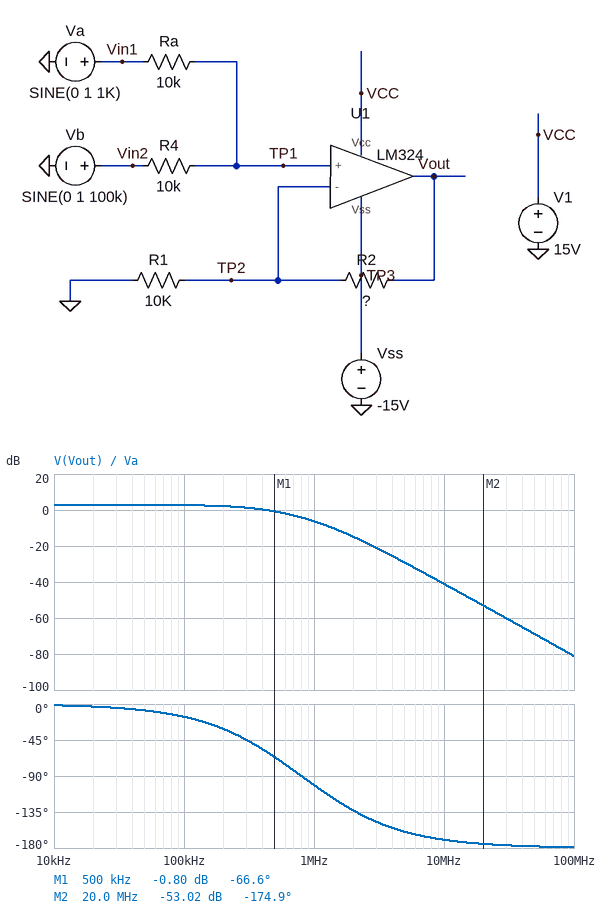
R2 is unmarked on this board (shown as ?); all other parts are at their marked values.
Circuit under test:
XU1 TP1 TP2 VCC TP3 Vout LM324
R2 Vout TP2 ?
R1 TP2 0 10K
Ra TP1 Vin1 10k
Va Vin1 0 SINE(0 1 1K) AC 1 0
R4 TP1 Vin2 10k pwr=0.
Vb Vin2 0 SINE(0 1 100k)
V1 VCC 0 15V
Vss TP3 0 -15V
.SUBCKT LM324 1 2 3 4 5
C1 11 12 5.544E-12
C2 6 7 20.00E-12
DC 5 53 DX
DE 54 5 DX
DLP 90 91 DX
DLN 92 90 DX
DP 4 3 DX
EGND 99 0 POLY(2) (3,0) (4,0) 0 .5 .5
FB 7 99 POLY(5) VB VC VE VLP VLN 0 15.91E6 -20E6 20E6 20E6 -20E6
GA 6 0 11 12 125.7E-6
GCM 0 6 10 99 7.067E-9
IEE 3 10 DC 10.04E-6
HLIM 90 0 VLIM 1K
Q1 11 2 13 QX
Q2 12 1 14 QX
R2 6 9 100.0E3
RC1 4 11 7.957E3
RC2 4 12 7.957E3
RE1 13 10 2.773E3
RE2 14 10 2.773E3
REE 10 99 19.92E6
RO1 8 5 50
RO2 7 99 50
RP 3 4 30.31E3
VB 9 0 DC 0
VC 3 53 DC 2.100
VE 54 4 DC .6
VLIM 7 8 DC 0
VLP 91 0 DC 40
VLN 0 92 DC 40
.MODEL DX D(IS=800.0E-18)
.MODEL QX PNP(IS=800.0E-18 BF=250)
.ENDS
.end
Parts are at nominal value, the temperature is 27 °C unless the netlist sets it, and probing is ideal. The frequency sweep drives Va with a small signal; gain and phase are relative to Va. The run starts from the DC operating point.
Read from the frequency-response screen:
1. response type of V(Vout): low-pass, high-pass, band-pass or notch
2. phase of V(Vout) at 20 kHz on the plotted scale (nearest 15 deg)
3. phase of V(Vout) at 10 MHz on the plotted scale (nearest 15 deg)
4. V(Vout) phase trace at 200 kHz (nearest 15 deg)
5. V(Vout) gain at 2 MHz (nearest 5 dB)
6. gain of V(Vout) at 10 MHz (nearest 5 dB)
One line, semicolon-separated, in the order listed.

low-pass; 0 deg; -165 deg; -30 deg; -15 dB; -40 dB
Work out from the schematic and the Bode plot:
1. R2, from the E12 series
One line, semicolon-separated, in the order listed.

18 kΩ
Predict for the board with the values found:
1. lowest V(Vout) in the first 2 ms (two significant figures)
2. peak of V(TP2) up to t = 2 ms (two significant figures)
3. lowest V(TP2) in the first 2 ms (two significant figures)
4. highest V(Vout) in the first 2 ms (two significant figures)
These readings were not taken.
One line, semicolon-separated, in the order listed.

-2.5 V; 900 mV; -900 mV; 2.5 V
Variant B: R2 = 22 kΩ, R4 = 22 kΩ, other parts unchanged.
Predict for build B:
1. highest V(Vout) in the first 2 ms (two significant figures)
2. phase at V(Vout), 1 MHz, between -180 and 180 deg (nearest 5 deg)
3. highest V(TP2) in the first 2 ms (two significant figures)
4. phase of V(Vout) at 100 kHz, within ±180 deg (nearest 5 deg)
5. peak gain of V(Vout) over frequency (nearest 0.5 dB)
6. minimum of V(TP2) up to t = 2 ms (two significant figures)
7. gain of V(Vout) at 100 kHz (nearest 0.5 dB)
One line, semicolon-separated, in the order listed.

3.1 V; -105 deg; 980 mV; -20 deg; 7.0 dB; -980 mV; 6.5 dB
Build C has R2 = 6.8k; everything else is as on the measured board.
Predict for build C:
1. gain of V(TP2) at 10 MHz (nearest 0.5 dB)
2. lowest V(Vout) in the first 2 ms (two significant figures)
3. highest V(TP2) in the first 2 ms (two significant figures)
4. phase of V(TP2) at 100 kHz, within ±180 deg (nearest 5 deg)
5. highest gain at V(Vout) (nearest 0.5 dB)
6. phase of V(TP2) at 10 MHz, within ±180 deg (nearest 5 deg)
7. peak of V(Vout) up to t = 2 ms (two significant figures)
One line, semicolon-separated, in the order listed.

-46.5 dB; -1.7 V; 1.0 V; -10 deg; -1.5 dB; -170 deg; 1.7 V
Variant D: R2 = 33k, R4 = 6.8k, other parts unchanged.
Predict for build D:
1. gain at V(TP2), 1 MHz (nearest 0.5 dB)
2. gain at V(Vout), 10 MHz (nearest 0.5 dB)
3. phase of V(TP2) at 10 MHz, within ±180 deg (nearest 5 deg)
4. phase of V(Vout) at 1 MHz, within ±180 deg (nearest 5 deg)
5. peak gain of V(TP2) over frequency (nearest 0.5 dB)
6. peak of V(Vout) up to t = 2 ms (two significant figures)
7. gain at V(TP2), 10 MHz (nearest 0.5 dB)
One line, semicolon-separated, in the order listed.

-21.0 dB; -43.0 dB; -160 deg; -110 deg; -8.0 dB; 2.9 V; -61.0 dB
